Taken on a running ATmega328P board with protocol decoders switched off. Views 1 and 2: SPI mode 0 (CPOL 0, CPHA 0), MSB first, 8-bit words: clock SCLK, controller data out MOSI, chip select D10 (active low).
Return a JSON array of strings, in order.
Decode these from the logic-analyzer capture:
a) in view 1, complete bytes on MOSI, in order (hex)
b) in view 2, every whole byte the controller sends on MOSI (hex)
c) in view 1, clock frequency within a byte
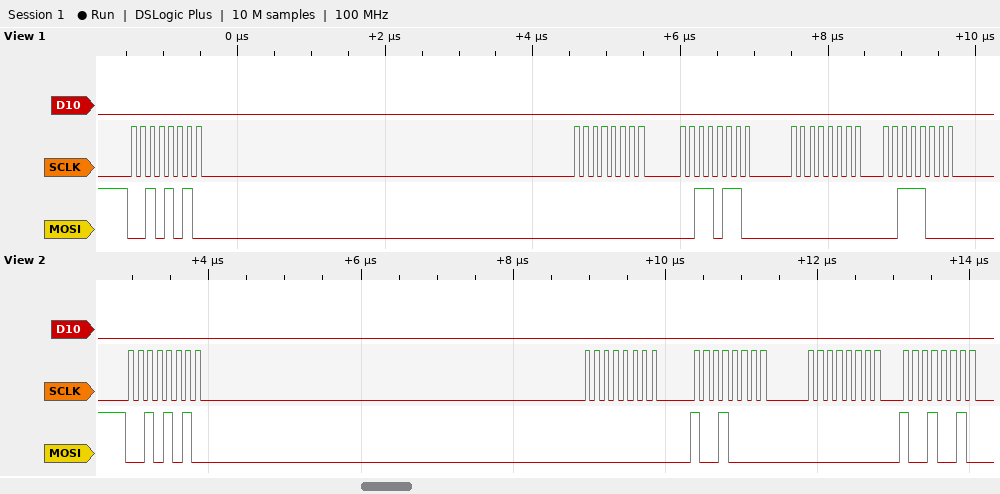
["2A 00 36 00 38", "0x2A 0x00 0x90 0x00 0x92", "8 MHz"]
